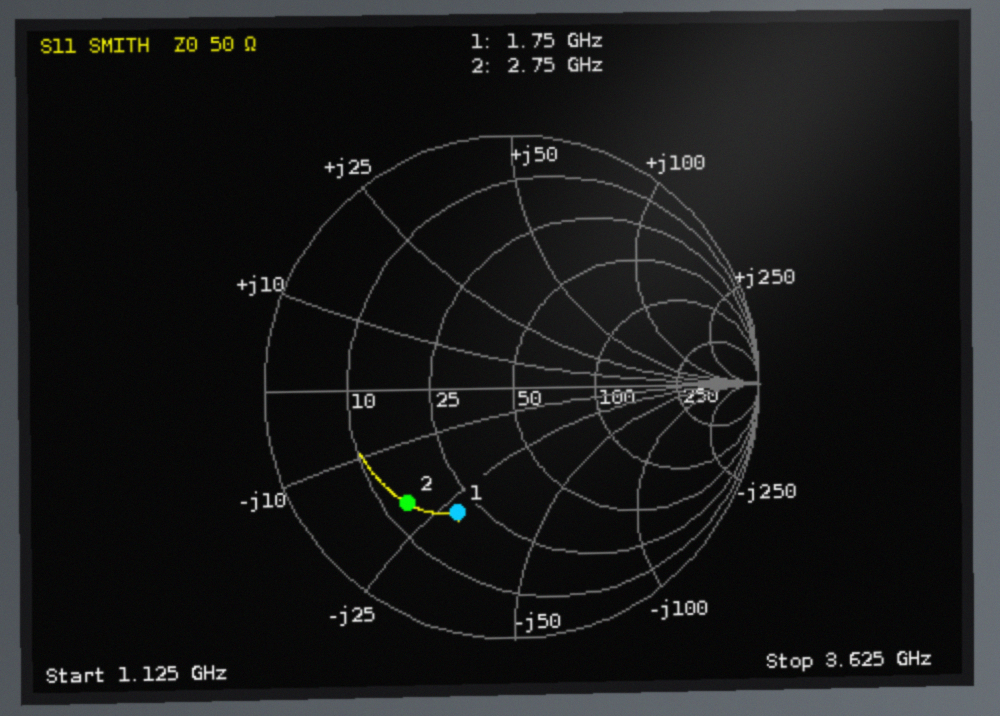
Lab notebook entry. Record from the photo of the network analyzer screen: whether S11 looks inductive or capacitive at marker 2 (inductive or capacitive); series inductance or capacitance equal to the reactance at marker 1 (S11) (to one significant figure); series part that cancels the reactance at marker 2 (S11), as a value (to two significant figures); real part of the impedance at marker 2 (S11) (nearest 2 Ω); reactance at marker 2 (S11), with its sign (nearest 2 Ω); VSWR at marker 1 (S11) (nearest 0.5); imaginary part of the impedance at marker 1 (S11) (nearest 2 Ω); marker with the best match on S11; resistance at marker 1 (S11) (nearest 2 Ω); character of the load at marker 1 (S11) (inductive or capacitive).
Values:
capacitive
3 pF
1.2 nH
14 Ω
-20 Ω
3.5
-28 Ω
marker 1
20 Ω
capacitive
